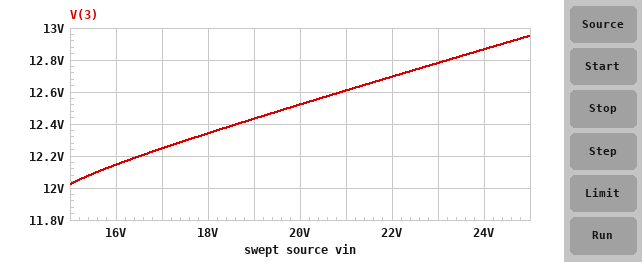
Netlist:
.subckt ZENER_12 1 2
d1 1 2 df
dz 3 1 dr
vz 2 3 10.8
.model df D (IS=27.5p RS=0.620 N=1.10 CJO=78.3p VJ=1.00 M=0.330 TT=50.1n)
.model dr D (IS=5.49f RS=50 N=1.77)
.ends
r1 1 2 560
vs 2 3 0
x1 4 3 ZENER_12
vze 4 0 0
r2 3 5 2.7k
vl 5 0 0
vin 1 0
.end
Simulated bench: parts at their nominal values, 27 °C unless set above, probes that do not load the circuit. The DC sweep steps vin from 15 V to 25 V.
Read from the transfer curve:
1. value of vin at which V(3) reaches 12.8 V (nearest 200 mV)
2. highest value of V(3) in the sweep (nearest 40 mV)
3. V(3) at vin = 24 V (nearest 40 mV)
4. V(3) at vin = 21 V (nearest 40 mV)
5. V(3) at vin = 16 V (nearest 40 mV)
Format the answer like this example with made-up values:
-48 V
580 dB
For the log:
23.2 V
12.96 V
12.88 V
12.60 V
12.16 V
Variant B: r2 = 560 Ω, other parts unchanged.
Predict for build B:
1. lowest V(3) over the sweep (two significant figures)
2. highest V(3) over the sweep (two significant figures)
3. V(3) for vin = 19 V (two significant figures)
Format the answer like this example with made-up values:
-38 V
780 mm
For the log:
7.5 V
12 V
9.5 V
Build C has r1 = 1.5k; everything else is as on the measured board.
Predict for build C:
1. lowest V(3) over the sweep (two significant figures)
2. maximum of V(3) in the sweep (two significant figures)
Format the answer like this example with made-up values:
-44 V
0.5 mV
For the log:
9.6 V
12 V
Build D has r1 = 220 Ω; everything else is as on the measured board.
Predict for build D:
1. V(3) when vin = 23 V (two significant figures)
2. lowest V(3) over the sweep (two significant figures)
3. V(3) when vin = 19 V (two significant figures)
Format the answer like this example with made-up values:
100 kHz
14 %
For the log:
14 V
12 V
13 V
